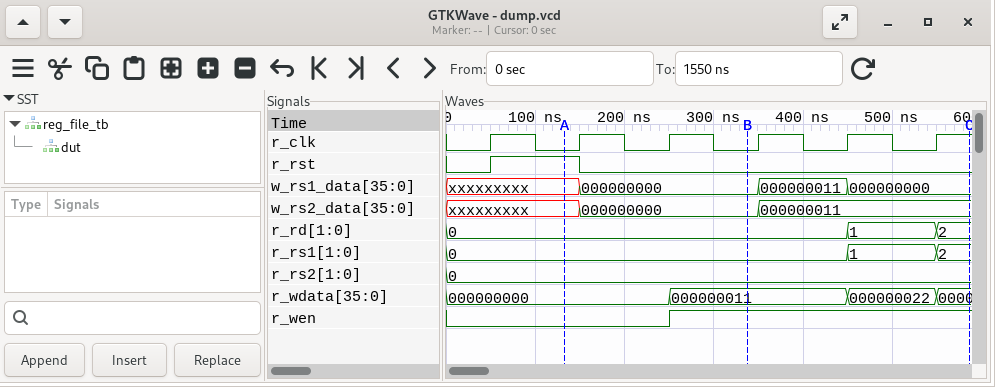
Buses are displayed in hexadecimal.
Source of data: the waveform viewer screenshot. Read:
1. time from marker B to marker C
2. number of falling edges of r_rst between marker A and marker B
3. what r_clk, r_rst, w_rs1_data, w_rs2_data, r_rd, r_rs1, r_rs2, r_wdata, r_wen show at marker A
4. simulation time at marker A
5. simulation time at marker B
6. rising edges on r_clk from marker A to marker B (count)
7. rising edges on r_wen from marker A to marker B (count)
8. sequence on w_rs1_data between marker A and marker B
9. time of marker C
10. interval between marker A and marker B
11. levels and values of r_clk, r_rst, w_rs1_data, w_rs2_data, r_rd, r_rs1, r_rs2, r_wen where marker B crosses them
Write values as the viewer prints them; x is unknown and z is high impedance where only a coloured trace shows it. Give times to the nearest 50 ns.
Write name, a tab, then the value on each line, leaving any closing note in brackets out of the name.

time from marker B to marker C	250 ns
number of falling edges of r_rst between marker A and marker B	1
what r_clk, r_rst, w_rs1_data, w_rs2_data, r_rd, r_rs1, r_rs2, r_wdata, r_wen show at marker A	r_clk=0, r_rst=1, w_rs1_data=xxxxxxxxx, w_rs2_data=xxxxxxxxx, r_rd=0, r_rs1=0, r_rs2=0, r_wdata=000000000, r_wen=0
simulation time at marker A	150 ns
simulation time at marker B	350 ns
rising edges on r_clk from marker A to marker B	2
rising edges on r_wen from marker A to marker B	1
sequence on w_rs1_data between marker A and marker B	xxxxxxxxx, 000000000
time of marker C	600 ns
interval between marker A and marker B	200 ns
levels and values of r_clk, r_rst, w_rs1_data, w_rs2_data, r_rd, r_rs1, r_rs2, r_wen where marker B crosses them	r_clk=0, r_rst=0, w_rs1_data=000000000, w_rs2_data=000000000, r_rd=0, r_rs1=0, r_rs2=0, r_wen=1
